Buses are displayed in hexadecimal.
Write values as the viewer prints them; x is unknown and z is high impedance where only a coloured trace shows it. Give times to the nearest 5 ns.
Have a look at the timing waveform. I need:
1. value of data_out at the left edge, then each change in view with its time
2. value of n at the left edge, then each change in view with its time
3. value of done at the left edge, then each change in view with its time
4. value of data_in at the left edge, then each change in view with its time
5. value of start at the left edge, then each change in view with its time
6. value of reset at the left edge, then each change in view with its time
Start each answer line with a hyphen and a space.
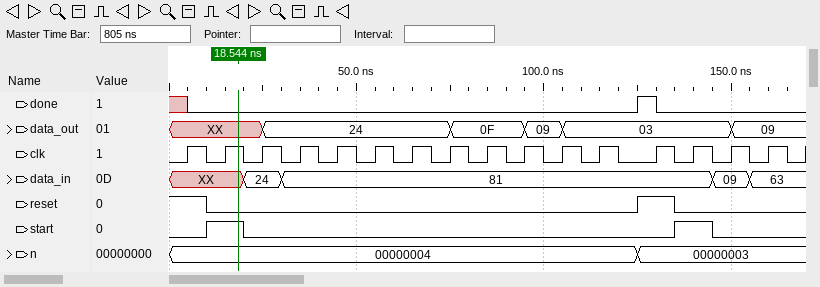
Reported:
- XX, 24 at 25 ns, 0F at 75 ns, 09 at 95 ns, 03 at 105 ns, 09 at 150 ns
- 00000004, 00000003 at 125 ns
- x, 0 at 5 ns, 1 at 125 ns, 0 at 130 ns
- XX, 24 at 20 ns, 81 at 30 ns, 09 at 145 ns, 63 at 155 ns
- 0, 1 at 10 ns, 0 at 20 ns, 1 at 135 ns, 0 at 145 ns
- 1, 0 at 10 ns, 1 at 125 ns, 0 at 135 ns
